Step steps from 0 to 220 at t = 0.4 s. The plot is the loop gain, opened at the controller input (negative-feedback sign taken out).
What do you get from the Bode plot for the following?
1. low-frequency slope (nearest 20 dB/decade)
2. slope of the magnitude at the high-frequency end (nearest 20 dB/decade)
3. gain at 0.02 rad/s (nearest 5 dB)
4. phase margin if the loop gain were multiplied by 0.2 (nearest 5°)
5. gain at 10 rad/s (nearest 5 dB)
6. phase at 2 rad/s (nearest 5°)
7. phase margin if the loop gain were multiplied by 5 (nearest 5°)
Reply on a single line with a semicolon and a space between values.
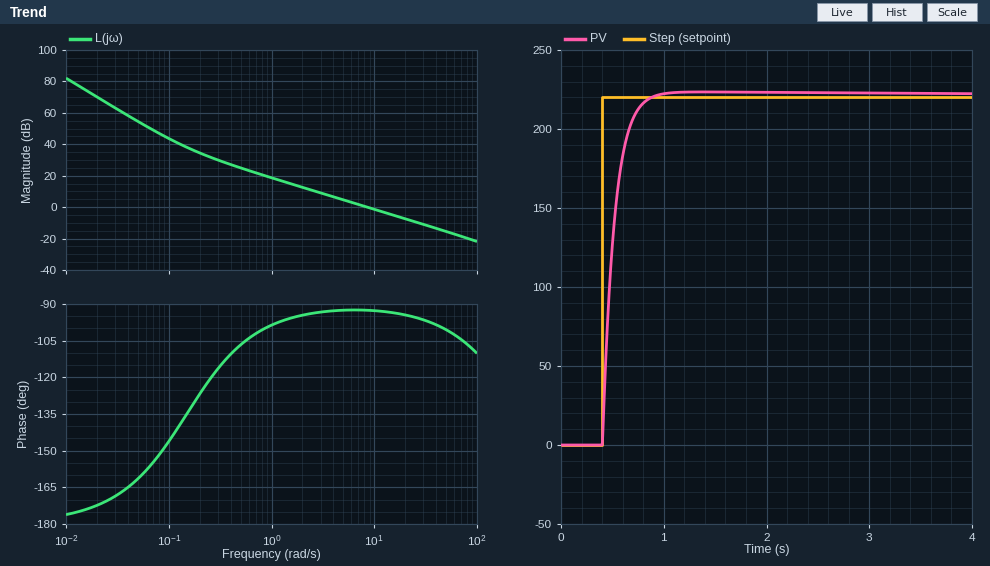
-40 dB/decade; -20 dB/decade; 70 dB; 85°; 0 dB; -95°; 80°
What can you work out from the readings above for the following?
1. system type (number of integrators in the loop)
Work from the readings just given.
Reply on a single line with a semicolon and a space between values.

2
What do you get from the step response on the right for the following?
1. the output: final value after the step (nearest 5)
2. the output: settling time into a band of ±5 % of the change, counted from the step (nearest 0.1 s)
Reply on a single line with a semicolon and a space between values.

220; 0.3 s
